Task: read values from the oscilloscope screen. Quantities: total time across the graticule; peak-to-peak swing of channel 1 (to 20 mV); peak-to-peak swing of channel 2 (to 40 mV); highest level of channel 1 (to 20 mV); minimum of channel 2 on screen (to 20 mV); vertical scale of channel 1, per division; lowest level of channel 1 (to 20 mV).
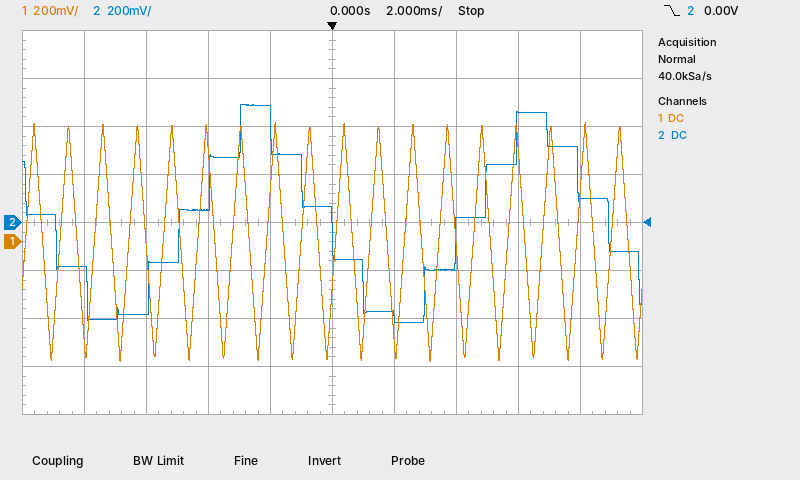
20 ms
1.00 V
920 mV
500 mV
-420 mV
200 mV
-500 mV
